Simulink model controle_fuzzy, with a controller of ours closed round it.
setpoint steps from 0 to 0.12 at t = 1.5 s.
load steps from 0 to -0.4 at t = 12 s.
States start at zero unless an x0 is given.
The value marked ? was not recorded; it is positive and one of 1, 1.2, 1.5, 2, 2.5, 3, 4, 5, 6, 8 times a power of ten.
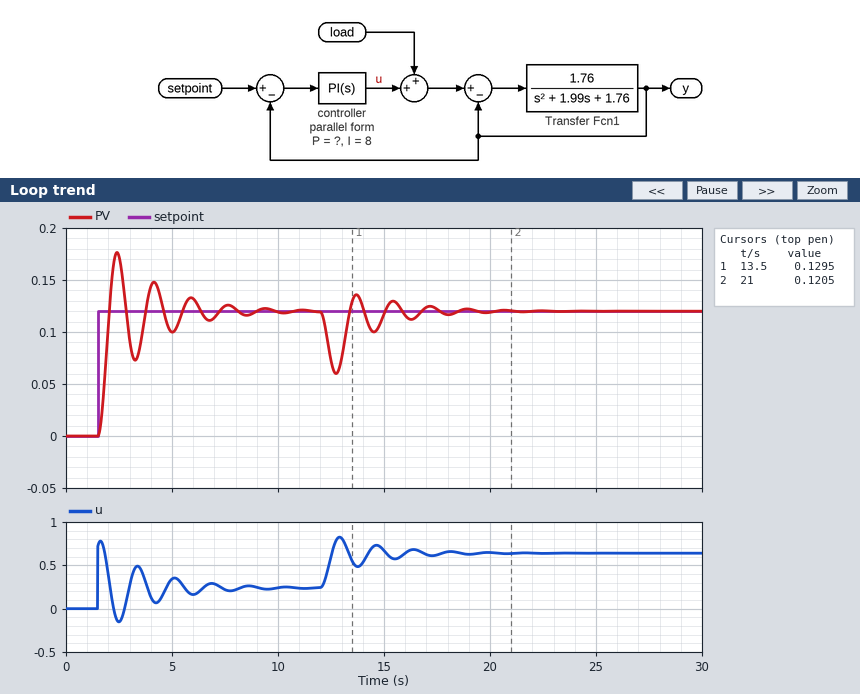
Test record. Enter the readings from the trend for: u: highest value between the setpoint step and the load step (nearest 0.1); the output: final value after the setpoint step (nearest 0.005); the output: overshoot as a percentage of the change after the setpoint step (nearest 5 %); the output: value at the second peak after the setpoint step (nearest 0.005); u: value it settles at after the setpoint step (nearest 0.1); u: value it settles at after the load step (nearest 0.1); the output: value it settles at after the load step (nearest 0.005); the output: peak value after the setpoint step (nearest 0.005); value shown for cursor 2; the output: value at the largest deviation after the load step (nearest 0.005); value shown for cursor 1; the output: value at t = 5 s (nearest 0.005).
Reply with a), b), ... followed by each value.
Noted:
a) 0.8
b) 0.120
c) 45 %
d) 0.150
e) 0.2
f) 0.6
g) 0.120
h) 0.175
i) 0.1205
j) 0.060
k) 0.1295
l) 0.100
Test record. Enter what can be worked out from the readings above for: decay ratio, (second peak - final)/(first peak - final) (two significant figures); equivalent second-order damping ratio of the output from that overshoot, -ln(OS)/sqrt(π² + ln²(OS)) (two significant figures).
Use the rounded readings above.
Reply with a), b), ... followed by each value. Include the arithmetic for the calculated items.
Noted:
a) (0.15 - 0.12) / (0.175 - 0.12) = 0.55
b) ln(0.45) = -0.799; 0.799 / sqrt(9.870 + 0.638) = 0.25
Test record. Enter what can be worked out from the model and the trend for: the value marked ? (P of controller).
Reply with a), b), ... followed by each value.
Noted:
a) 6
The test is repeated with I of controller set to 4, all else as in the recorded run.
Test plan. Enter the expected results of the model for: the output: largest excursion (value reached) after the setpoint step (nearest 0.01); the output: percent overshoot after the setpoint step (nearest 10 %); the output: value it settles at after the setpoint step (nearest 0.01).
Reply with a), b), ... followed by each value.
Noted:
a) 0.15
b) 30 %
c) 0.12
